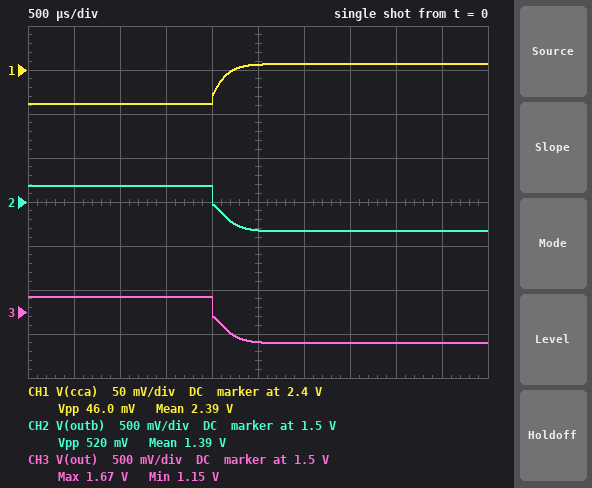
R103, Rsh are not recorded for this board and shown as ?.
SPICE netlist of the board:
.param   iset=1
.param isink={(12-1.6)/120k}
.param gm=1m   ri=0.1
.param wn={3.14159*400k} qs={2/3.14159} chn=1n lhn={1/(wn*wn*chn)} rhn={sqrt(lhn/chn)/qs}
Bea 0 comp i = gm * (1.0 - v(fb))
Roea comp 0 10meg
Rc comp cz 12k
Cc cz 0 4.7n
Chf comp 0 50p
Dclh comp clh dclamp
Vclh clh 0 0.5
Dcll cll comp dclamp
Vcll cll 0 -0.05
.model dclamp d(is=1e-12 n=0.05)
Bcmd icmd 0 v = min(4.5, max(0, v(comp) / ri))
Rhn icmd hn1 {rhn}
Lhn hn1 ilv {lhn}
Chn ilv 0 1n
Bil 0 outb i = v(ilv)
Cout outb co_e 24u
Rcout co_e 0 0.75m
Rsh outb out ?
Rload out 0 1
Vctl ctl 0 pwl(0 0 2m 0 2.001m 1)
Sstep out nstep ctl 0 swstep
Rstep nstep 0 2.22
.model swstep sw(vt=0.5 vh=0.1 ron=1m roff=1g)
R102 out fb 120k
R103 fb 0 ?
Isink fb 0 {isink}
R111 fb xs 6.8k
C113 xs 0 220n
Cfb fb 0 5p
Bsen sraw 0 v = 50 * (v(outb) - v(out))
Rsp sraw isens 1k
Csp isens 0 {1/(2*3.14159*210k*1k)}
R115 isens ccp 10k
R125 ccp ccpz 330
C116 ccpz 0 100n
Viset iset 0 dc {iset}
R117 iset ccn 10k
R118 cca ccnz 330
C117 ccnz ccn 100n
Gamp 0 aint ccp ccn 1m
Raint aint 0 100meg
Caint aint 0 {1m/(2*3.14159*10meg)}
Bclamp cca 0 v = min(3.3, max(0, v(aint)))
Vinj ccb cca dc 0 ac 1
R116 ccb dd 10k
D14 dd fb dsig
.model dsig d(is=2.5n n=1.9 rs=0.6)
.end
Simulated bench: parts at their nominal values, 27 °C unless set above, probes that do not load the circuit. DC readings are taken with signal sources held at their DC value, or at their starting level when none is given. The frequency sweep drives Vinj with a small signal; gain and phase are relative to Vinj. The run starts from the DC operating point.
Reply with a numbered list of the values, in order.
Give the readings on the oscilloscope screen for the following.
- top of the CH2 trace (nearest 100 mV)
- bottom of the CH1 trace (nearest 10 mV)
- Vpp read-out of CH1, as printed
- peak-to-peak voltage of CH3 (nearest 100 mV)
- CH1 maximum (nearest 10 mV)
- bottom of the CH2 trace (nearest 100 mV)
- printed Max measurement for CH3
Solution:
1. 1.7 V
2. 2.36 V
3. 46.0 mV
4. 500 mV
5. 2.41 V
6. 1.2 V
7. 1.67 V
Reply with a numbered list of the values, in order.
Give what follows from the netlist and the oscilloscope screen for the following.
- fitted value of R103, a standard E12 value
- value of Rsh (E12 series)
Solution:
1. 270 kΩ
2. 0.012 Ω
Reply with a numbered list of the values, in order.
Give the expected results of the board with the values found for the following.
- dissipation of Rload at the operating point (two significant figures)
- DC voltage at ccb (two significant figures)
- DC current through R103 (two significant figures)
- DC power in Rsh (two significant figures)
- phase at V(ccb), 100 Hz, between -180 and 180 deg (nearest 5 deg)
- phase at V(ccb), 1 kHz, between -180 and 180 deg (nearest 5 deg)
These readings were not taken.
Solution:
1. 2.8 W
2. 2.4 V
3. 3.7 µA
4. 33 mW
5. 85 deg
6. 40 deg
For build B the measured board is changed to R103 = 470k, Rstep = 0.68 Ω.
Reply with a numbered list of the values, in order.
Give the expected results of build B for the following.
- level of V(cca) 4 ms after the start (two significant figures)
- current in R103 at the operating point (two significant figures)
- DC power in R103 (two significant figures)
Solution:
1. 2.4 V
2. 2.1 µA
3. 2.1 µW
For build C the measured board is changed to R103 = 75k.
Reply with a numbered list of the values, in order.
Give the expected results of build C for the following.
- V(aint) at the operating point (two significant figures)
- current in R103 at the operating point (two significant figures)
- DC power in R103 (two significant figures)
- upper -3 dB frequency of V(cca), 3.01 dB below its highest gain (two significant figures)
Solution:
1. 2.5 V
2. 13 µA
3. 13 µW
4. 920 Hz
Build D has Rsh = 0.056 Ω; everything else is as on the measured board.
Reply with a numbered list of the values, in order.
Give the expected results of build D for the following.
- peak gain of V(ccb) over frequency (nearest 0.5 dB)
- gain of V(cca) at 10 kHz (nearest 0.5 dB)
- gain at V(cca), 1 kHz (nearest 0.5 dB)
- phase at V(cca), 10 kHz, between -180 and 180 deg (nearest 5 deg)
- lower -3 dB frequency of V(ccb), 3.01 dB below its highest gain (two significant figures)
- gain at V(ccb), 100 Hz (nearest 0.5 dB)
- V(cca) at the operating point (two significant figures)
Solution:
1. 2.5 dB
2. -5.5 dB
3. -0.5 dB
4. 155 deg
5. 45 kHz
6. -34.0 dB
7. 2.5 V
